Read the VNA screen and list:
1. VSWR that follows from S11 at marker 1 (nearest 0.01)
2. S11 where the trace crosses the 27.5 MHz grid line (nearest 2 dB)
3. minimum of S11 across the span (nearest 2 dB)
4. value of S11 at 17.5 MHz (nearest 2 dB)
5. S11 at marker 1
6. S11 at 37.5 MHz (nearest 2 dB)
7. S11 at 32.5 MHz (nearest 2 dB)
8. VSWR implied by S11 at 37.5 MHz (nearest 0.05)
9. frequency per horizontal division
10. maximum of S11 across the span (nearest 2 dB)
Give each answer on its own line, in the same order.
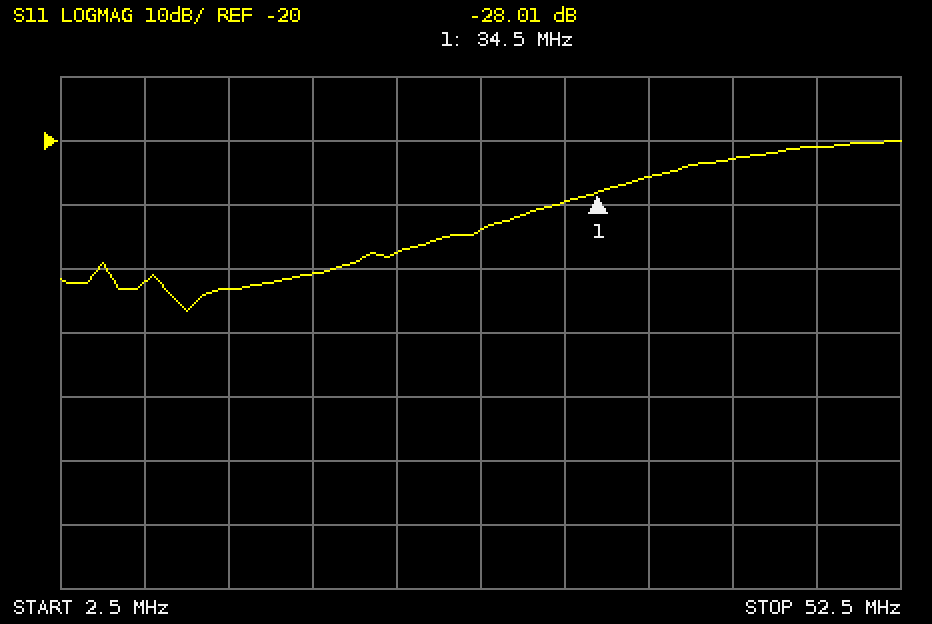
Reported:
1.08
-34 dB
-46 dB
-40 dB
-28.01 dB
-26 dB
-30 dB
1.10
5 MHz
-20 dB
